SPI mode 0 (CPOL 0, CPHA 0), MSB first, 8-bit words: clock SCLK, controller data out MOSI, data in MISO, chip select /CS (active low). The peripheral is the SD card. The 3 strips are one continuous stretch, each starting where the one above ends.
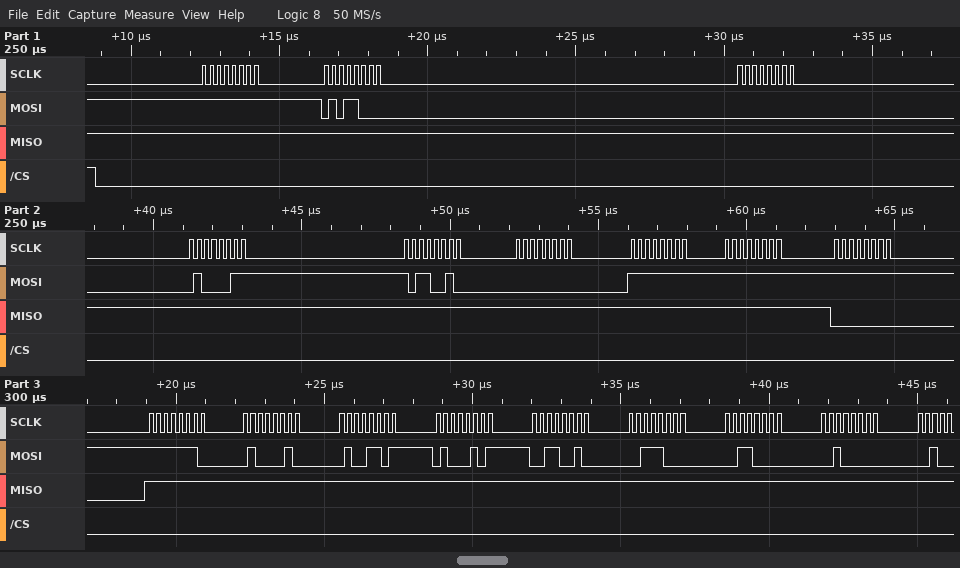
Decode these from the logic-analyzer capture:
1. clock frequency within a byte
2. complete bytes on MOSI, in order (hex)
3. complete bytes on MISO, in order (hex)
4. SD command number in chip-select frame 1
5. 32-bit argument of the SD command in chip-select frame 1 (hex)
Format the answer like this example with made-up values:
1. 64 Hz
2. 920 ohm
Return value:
1. 4 MHz
2. FF 58 00 43 B2 00 FF FF FF FE 42 4D 45 32 38 30 20
3. FF FF FF FF FF FF FF FF 00 FF FF FF FF FF FF FF FF
4. CMD24
5. 0x0043B200
